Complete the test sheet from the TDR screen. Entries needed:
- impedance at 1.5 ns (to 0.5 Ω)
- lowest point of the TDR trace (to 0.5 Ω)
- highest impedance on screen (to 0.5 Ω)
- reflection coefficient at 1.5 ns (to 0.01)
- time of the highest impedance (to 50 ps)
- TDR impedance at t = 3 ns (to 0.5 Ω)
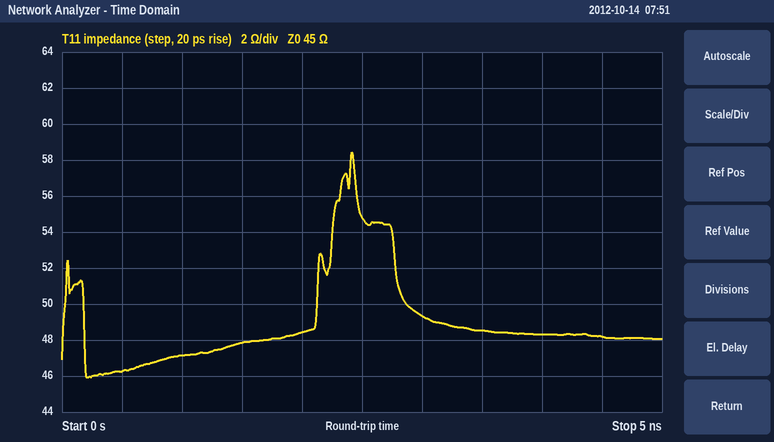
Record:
48.0 Ω
46.0 Ω
58.5 Ω
+0.03
2.40 ns
49.5 Ω
